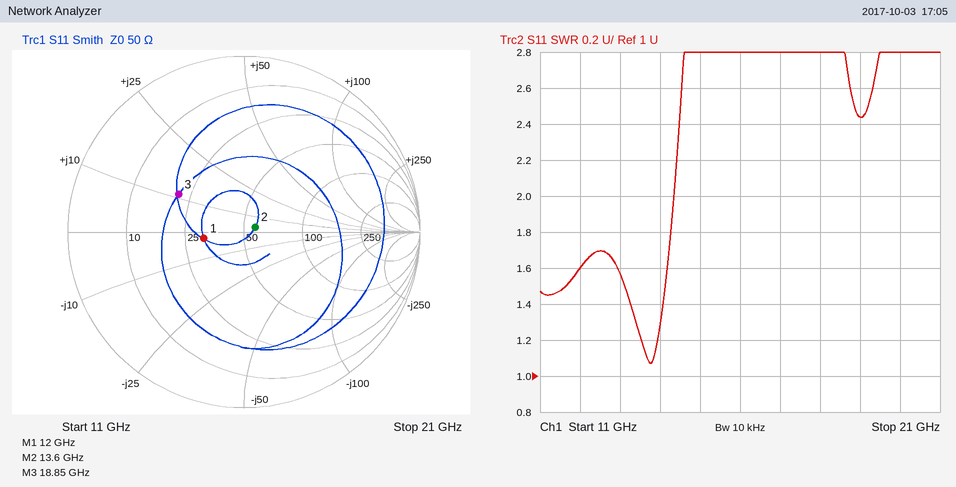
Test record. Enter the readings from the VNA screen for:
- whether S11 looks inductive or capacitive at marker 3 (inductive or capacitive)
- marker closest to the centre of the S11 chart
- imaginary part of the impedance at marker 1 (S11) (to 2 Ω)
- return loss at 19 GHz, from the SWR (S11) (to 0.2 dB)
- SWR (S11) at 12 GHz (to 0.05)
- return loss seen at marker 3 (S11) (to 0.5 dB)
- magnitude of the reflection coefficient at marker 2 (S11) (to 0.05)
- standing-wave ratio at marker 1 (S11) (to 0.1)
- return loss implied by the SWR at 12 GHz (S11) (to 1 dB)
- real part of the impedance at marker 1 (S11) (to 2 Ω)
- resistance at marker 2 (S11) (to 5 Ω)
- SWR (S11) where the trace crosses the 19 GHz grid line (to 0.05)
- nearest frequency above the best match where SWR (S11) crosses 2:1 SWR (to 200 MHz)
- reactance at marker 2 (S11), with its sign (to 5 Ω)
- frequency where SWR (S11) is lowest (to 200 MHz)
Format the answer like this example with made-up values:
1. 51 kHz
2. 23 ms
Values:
1. inductive
2. marker 2
3. -2 Ω
4. 7.6 dB
5. 1.60
6. 7.5 dB
7. 0.05
8. 1.6
9. 13 dB
10. 32 Ω
11. 55 Ω
12. 2.45
13. 14.4 GHz
14. +5 Ω
15. 13.8 GHz
